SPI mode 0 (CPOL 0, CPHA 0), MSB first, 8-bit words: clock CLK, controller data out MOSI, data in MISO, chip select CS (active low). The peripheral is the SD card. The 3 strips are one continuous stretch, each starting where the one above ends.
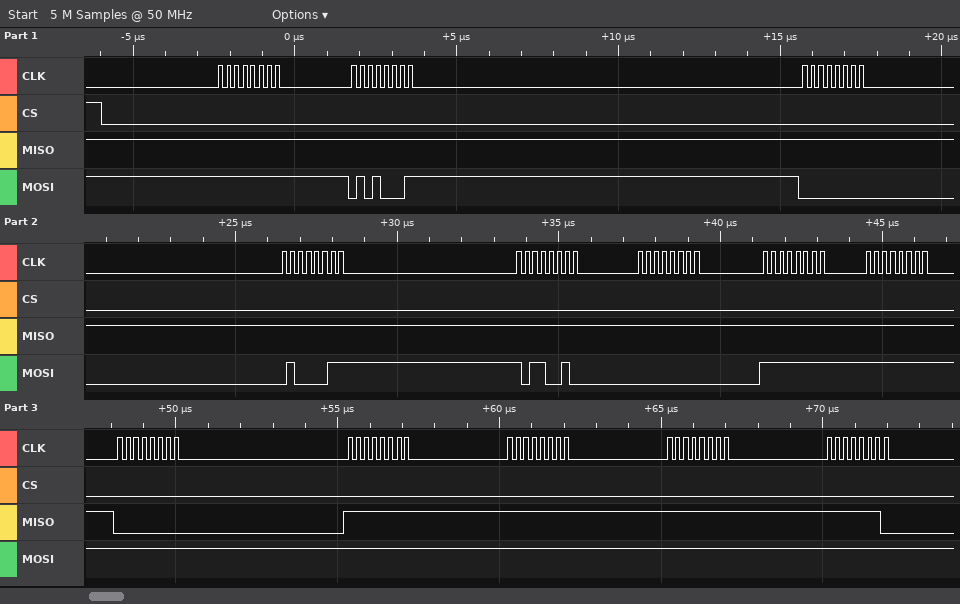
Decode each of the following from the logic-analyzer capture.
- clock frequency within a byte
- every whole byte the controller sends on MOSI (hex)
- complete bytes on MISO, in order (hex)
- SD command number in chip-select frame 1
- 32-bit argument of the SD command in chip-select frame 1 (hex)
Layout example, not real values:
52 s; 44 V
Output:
4 MHz; FF 51 00 43 B2 00 FF FF FF FF FF FF FF; FF FF FF FF FF FF FF FF 00 FF FF FF FE; CMD17; 0x0043B200
